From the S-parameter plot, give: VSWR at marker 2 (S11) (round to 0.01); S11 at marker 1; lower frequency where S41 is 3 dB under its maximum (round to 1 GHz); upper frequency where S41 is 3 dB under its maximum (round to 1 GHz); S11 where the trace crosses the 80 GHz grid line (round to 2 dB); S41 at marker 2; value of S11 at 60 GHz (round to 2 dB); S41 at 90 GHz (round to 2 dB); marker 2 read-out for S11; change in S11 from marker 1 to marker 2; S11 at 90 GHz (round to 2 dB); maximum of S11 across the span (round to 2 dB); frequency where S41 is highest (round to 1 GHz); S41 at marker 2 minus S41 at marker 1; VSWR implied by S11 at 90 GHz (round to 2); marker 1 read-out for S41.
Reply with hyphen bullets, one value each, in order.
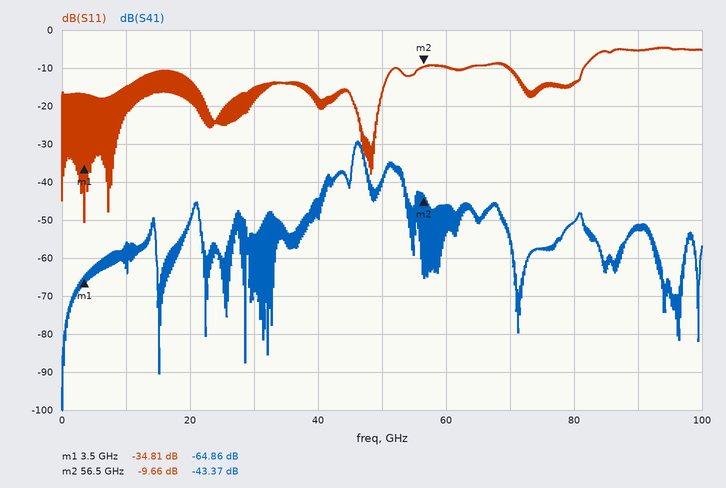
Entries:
- 1.98
- -34.81 dB
- 46 GHz
- 47 GHz
- -14 dB
- -43.37 dB
- -10 dB
- -52 dB
- -9.66 dB
- 25.15 dB
- -6 dB
- -4 dB
- 46 GHz
- 21.49 dB
- 4
- -64.86 dB
